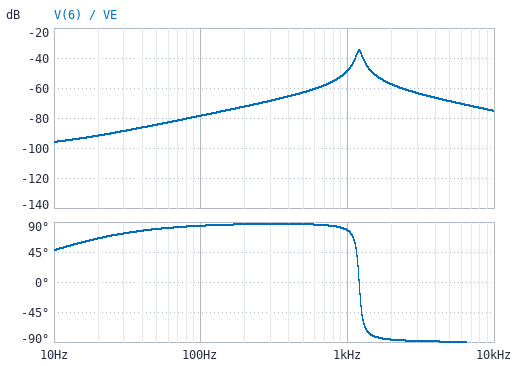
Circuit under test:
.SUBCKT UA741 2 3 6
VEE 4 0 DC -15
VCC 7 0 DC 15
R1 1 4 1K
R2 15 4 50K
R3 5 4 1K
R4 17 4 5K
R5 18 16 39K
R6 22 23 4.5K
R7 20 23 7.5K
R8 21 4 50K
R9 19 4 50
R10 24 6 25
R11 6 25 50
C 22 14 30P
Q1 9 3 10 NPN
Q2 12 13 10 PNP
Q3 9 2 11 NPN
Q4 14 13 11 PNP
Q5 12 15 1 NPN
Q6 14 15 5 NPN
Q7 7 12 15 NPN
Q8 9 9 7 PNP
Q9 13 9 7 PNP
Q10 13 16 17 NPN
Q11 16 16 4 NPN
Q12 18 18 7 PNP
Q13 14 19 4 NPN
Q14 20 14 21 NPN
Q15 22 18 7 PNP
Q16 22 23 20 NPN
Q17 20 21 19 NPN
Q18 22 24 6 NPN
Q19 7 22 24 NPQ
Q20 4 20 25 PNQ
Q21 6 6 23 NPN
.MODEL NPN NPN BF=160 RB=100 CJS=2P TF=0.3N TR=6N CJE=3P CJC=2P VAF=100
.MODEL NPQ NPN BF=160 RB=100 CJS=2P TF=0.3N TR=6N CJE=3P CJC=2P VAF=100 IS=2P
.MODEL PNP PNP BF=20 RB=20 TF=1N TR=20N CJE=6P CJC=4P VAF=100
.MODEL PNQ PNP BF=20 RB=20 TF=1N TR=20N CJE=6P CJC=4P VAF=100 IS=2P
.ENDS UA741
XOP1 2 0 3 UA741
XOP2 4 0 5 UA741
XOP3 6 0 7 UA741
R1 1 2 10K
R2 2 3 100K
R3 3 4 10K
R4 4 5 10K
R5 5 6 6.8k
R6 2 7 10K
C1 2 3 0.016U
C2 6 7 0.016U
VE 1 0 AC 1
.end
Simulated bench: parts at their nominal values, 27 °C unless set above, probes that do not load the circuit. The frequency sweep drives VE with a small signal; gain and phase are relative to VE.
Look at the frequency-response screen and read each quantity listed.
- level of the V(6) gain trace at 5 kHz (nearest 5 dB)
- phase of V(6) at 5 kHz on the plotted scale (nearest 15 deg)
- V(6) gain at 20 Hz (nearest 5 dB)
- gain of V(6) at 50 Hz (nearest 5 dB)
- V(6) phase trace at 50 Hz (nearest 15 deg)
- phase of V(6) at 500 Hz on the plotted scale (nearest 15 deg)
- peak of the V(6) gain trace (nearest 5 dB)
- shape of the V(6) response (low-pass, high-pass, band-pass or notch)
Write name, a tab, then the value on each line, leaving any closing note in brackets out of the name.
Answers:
level of the V(6) gain trace at 5 kHz	-70 dB
phase of V(6) at 5 kHz on the plotted scale	-90 deg
V(6) gain at 20 Hz	-90 dB
gain of V(6) at 50 Hz	-85 dB
V(6) phase trace at 50 Hz	75 deg
phase of V(6) at 500 Hz on the plotted scale	90 deg
peak of the V(6) gain trace	-35 dB
shape of the V(6) response	band-pass
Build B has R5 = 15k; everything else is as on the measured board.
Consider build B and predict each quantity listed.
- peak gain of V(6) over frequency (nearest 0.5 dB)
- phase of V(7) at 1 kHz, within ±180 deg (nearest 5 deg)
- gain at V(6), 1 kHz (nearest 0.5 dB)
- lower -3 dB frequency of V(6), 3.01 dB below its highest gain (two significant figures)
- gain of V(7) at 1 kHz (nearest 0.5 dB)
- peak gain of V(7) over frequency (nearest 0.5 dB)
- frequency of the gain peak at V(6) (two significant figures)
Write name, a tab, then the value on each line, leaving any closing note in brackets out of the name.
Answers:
peak gain of V(6) over frequency	-42.0 dB
phase of V(7) at 1 kHz, within ±180 deg	15 deg
gain at V(6), 1 kHz	-53.0 dB
lower -3 dB frequency of V(6), 3.01 dB below its highest gain	760 Hz
gain of V(7) at 1 kHz	5.5 dB
peak gain of V(7) over frequency	18.5 dB
frequency of the gain peak at V(6)	810 Hz
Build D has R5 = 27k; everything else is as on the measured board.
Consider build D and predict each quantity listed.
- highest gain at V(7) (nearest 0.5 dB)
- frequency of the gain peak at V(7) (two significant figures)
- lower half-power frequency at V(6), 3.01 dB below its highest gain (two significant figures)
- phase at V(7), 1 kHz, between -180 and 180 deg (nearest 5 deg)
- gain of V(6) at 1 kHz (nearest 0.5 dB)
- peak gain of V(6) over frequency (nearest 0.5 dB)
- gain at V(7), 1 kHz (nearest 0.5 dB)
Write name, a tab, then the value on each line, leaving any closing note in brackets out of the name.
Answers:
highest gain at V(7)	16.0 dB
frequency of the gain peak at V(7)	600 Hz
lower half-power frequency at V(6), 3.01 dB below its highest gain	560 Hz
phase at V(7), 1 kHz, between -180 and 180 deg	10 deg
gain of V(6) at 1 kHz	-63.5 dB
peak gain of V(6) over frequency	-47.0 dB
gain at V(7), 1 kHz	-5.0 dB
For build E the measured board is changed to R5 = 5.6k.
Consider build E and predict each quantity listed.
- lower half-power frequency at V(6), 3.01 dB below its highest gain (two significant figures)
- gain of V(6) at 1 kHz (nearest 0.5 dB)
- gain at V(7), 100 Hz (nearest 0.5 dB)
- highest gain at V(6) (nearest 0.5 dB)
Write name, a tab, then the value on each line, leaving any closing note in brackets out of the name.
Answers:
lower half-power frequency at V(6), 3.01 dB below its highest gain	1.3 kHz
gain of V(6) at 1 kHz	-51.5 dB
gain at V(7), 100 Hz	0 dB
highest gain at V(6)	-33.0 dB
